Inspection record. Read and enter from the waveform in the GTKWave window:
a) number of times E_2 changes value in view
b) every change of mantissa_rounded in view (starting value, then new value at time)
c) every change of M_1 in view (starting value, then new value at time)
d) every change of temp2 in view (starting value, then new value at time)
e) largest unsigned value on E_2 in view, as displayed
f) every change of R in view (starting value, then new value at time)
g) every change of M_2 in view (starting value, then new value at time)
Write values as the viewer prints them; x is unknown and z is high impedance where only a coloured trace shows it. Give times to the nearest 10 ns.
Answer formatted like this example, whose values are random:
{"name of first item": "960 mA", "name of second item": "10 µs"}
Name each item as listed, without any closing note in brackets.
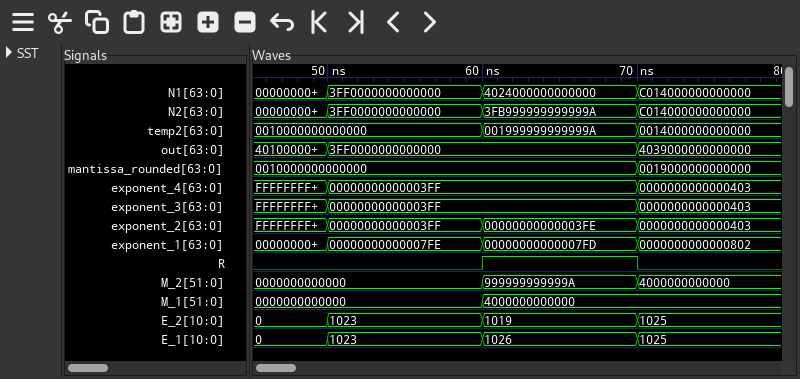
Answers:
{"number of times E_2 changes value in view": "3", "every change of mantissa_rounded in view": "0010000000000000, 0019000000000000 at 70 ns", "every change of M_1 in view": "0000000000000, 4000000000000 at 60 ns", "every change of temp2 in view": "0010000000000000, 001999999999999A at 60 ns, 0014000000000000 at 70 ns", "largest unsigned value on E_2 in view, as displayed": "1025", "every change of R in view": "0, 1 at 60 ns, 0 at 70 ns", "every change of M_2 in view": "0000000000000, 999999999999A at 60 ns, 4000000000000 at 70 ns"}
